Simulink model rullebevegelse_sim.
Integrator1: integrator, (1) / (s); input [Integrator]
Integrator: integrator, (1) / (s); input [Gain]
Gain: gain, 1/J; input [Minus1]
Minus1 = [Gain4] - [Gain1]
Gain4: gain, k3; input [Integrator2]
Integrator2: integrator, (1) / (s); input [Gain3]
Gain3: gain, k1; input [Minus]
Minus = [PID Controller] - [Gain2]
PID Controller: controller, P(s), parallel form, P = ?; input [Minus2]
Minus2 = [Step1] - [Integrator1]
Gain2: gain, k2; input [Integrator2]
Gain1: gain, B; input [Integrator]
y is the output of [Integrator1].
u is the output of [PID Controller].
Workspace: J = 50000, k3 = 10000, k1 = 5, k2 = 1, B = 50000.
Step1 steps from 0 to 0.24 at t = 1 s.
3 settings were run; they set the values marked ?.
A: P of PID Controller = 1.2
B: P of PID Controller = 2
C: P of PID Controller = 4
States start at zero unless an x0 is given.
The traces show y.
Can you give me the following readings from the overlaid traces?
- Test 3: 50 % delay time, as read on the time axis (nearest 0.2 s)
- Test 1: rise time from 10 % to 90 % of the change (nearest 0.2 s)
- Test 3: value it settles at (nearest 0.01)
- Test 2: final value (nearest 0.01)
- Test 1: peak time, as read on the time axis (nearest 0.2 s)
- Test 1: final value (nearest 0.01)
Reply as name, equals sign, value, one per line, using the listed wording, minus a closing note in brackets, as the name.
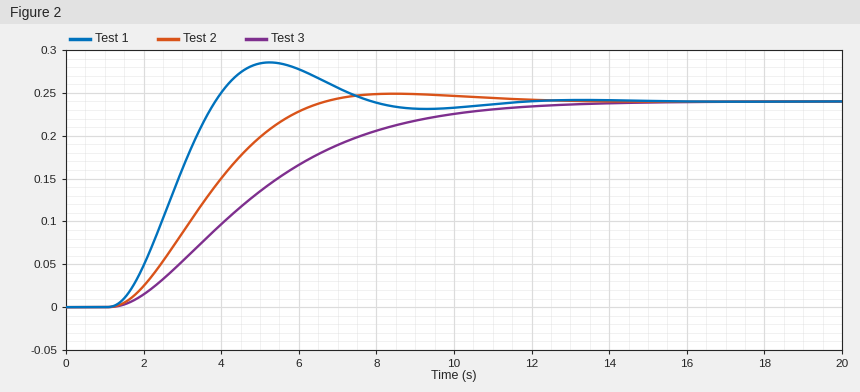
Test 3: 50 % delay time, as read on the time axis = 4.6 s
Test 1: rise time from 10 % to 90 % of the change = 1.8 s
Test 3: value it settles at = 0.24
Test 2: final value = 0.24
Test 1: peak time, as read on the time axis = 5.2 s
Test 1: final value = 0.24
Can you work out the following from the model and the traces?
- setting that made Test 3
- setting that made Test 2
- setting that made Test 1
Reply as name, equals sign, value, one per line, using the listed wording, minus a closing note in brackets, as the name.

setting that made Test 3 = A
setting that made Test 2 = B
setting that made Test 1 = C
